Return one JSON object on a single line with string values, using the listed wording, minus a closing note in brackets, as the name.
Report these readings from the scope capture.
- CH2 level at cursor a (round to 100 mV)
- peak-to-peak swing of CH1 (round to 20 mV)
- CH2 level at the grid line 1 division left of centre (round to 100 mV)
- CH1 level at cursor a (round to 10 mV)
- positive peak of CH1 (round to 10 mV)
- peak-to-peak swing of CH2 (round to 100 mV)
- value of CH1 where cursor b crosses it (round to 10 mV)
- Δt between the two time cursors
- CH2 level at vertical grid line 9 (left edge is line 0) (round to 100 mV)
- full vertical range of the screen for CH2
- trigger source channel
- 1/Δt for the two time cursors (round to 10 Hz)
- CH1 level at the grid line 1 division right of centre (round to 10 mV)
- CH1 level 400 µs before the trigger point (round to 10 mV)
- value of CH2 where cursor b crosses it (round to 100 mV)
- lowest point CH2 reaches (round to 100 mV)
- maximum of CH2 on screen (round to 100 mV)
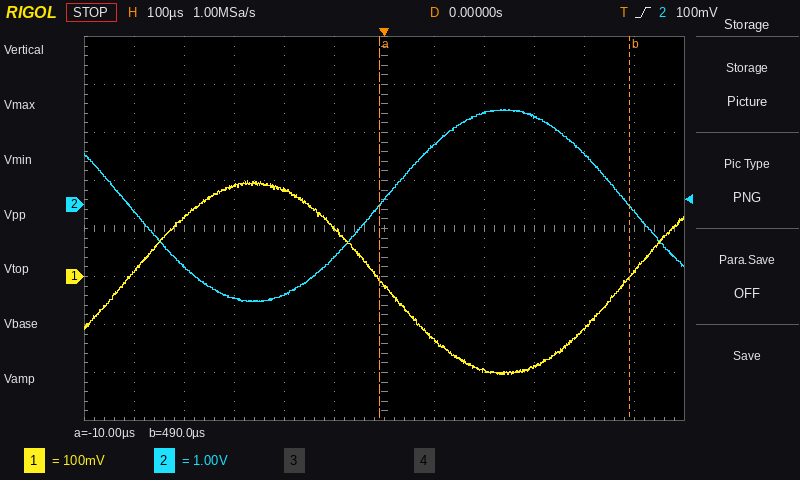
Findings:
{"CH2 level at cursor a": "0.0 V", "peak-to-peak swing of CH1": "400 mV", "CH2 level at the grid line 1 division left of centre": "-1.1 V", "CH1 level at cursor a": "-10 mV", "positive peak of CH1": "200 mV", "peak-to-peak swing of CH2": "4.0 V", "value of CH1 where cursor b crosses it": "0 mV", "Δt between the two time cursors": "500 µs", "CH2 level at vertical grid line 9 (left edge is line 0)": "1.8 V", "full vertical range of the screen for CH2": "8 V", "trigger source channel": "CH2", "1/Δt for the two time cursors": "2.00 kHz", "CH1 level at the grid line 1 division right of centre": "-130 mV", "CH1 level 400 µs before the trigger point": "120 mV", "value of CH2 where cursor b crosses it": "0.0 V", "lowest point CH2 reaches": "-2.0 V", "maximum of CH2 on screen": "2.0 V"}
